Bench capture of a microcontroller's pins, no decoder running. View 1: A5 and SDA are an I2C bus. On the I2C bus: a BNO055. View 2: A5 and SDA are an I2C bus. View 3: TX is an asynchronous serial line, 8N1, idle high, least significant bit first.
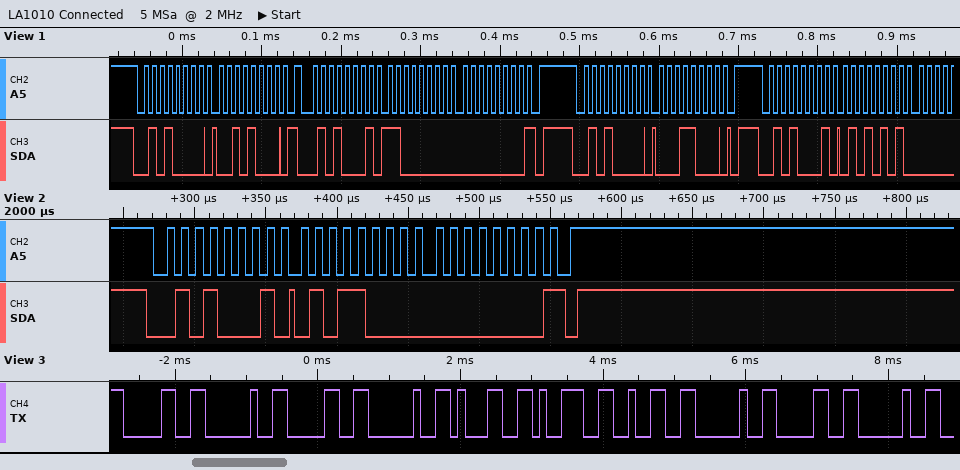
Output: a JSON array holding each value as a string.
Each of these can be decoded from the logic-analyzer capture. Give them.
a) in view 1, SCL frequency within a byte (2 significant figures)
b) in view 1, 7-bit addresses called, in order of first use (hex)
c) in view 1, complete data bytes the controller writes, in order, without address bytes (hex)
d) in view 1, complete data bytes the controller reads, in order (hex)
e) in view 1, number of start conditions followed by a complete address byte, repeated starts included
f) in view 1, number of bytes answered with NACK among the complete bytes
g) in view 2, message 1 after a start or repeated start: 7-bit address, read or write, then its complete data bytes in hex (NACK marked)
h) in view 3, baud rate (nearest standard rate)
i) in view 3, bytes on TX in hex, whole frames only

["100 kHz", "0x28", "28 18", "C0 00 55", "4", "1", "0x28 read: 58 00 NACK", "9600 baud", "30 20 30 20 31 39 32 20 30 20"]
